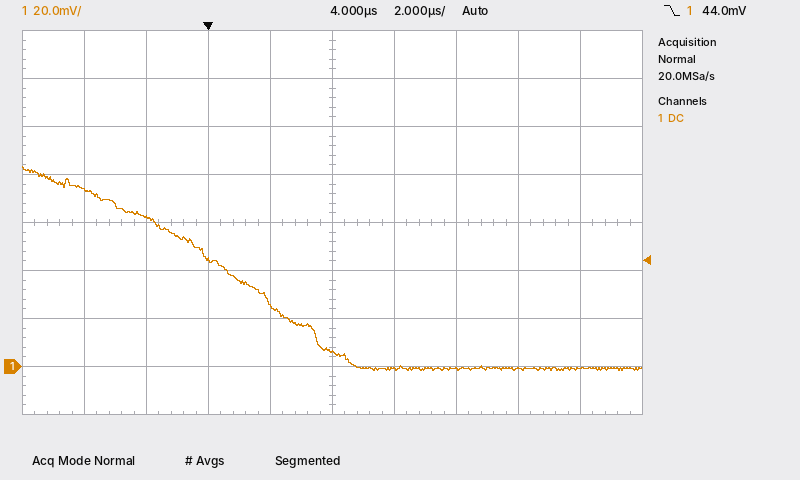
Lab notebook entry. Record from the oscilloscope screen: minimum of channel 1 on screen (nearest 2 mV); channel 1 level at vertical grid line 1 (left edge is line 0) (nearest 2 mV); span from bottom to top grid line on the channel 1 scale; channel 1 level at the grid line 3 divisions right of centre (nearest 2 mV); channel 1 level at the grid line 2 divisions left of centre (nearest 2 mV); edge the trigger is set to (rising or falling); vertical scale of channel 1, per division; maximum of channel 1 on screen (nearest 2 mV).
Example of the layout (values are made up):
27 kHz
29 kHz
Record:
-2 mV
74 mV
160 mV
0 mV
44 mV
falling
20 mV
84 mV
